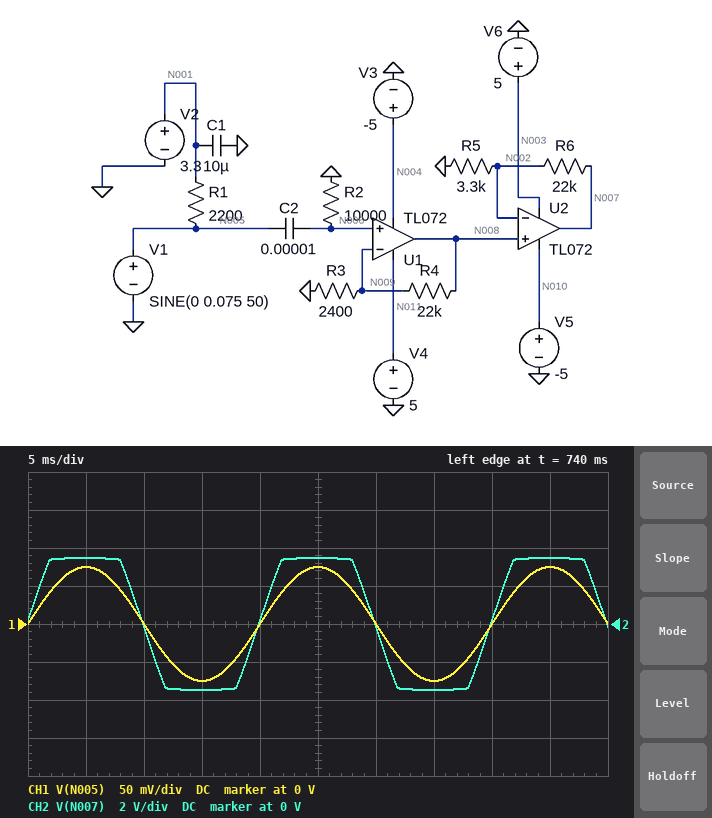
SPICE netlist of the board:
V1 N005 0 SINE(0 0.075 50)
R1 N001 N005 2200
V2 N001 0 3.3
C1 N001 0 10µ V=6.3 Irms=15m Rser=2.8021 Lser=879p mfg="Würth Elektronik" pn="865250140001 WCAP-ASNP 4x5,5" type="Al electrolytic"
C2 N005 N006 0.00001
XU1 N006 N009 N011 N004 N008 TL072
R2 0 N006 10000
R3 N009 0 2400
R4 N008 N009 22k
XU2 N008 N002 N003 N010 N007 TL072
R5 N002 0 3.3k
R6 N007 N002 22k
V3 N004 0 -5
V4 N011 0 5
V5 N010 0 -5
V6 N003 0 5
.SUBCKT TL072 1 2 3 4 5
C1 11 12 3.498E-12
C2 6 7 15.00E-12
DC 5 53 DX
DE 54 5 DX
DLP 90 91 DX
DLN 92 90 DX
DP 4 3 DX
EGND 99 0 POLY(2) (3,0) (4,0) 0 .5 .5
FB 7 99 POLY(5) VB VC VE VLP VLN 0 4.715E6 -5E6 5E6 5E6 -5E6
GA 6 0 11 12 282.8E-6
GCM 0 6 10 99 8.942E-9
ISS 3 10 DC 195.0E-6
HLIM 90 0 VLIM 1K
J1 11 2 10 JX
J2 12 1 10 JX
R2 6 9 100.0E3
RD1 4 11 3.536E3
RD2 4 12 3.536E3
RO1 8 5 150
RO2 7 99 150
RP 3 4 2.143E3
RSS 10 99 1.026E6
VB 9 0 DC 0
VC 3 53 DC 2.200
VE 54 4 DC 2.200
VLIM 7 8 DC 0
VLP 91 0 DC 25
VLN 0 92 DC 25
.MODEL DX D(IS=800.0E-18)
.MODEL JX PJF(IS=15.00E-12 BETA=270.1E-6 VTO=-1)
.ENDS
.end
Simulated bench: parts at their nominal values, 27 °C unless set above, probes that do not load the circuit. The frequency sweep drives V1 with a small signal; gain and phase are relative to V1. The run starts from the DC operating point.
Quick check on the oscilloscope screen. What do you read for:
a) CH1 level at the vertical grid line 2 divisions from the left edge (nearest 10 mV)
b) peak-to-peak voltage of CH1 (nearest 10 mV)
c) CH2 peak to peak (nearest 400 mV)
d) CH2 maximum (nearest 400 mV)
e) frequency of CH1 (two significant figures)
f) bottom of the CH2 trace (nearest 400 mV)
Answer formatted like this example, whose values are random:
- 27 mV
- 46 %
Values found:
- 0 V
- 150 mV
- 6.8 V
- 3.6 V
- 50 Hz
- -3.6 V
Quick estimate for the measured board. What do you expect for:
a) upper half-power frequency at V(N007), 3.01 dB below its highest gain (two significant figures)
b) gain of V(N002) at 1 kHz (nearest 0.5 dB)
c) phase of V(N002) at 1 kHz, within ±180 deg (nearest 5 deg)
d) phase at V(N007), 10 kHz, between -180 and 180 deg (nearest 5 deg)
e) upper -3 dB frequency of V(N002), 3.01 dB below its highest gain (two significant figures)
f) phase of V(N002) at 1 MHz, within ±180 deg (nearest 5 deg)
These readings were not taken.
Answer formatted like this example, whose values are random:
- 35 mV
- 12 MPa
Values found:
- 260 kHz
- 20.0 dB
- 0 deg
- -5 deg
- 260 kHz
- -155 deg
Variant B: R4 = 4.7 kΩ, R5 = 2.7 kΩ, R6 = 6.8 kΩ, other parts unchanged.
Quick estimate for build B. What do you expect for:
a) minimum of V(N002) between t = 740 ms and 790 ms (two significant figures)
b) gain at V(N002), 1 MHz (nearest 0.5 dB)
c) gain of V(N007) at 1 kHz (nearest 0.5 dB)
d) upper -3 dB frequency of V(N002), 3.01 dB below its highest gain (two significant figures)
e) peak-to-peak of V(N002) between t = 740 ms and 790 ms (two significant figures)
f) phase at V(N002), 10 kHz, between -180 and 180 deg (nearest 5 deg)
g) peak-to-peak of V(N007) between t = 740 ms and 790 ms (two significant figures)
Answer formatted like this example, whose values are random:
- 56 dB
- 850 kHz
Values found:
- -220 mV
- 5.0 dB
- 20.5 dB
- 810 kHz
- 440 mV
- 0 deg
- 1.6 V
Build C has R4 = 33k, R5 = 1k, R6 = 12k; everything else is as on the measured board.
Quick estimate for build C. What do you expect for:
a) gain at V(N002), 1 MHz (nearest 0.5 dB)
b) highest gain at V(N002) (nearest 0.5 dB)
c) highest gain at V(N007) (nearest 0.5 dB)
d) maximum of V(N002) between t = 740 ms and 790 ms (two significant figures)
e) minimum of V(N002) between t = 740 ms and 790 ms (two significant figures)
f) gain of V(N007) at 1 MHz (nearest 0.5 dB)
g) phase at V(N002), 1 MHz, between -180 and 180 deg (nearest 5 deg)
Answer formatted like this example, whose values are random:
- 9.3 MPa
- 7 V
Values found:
- -1.0 dB
- 23.5 dB
- 45.5 dB
- 270 mV
- -270 mV
- 21.5 dB
- -170 deg
